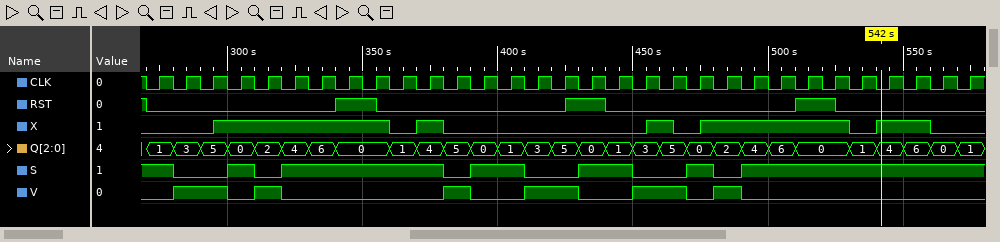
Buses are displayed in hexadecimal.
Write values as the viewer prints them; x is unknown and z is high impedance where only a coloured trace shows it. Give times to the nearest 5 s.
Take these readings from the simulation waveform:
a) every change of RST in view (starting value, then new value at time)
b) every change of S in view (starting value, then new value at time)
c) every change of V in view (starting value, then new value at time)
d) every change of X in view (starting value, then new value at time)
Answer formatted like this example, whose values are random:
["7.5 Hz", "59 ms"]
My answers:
["1, 0 at 270 s, 1 at 340 s, 0 at 355 s, 1 at 425 s, 0 at 440 s, 1 at 510 s, 0 at 525 s", "1, 0 at 280 s, 1 at 300 s, 0 at 310 s, 1 at 320 s, 0 at 380 s, 1 at 390 s, 0 at 410 s, 1 at 430 s, 0 at 450 s, 1 at 470 s, 0 at 480 s, 1 at 490 s", "0, 1 at 280 s, 0 at 300 s, 1 at 310 s, 0 at 320 s, 1 at 380 s, 0 at 390 s, 1 at 410 s, 0 at 430 s, 1 at 450 s, 0 at 470 s, 1 at 480 s, 0 at 490 s", "0, 1 at 295 s, 0 at 360 s, 1 at 370 s, 0 at 380 s, 1 at 455 s, 0 at 465 s, 1 at 475 s, 0 at 530 s, 1 at 540 s, 0 at 560 s"]
